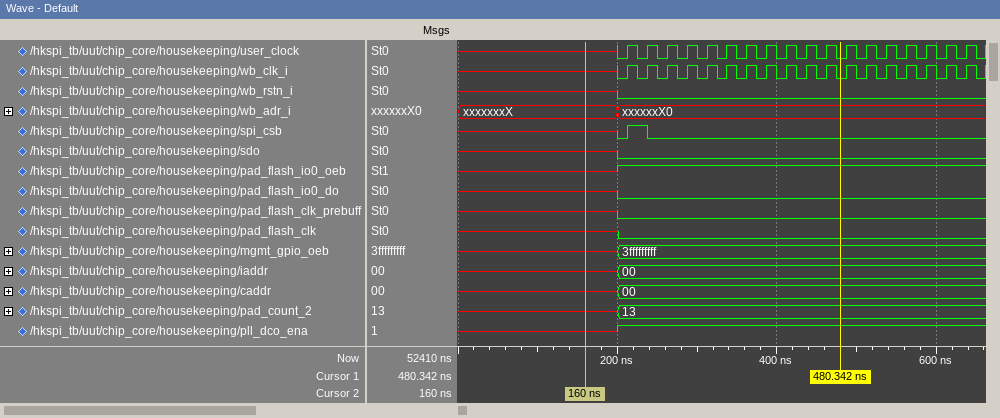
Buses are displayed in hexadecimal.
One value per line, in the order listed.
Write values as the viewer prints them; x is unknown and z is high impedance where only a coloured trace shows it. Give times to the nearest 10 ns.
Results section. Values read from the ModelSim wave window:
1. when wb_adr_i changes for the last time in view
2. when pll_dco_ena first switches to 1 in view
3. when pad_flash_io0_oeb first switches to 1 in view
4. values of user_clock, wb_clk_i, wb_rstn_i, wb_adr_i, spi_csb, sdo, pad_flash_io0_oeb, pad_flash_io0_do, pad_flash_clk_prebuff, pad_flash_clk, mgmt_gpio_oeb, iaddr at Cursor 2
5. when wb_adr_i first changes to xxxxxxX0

200 ns
200 ns
200 ns
user_clock=x, wb_clk_i=x, wb_rstn_i=x, wb_adr_i=xxxxxxxX, spi_csb=x, sdo=x, pad_flash_io0_oeb=x, pad_flash_io0_do=x, pad_flash_clk_prebuff=x, pad_flash_clk=x, mgmt_gpio_oeb=x, iaddr=x
200 ns
